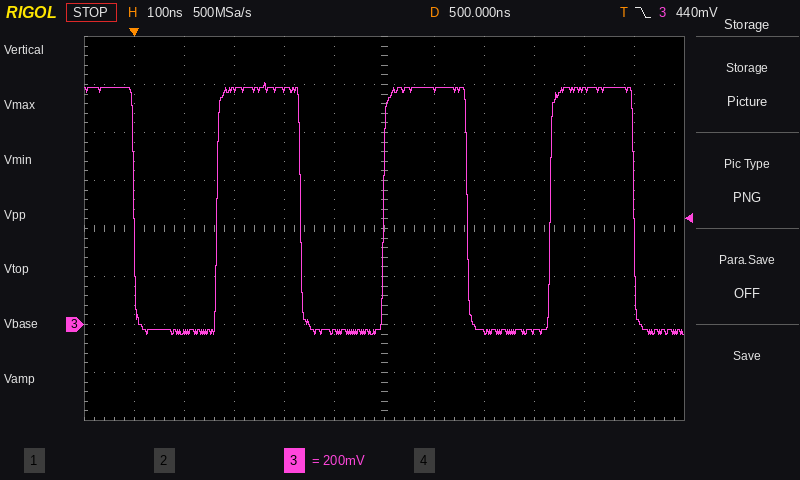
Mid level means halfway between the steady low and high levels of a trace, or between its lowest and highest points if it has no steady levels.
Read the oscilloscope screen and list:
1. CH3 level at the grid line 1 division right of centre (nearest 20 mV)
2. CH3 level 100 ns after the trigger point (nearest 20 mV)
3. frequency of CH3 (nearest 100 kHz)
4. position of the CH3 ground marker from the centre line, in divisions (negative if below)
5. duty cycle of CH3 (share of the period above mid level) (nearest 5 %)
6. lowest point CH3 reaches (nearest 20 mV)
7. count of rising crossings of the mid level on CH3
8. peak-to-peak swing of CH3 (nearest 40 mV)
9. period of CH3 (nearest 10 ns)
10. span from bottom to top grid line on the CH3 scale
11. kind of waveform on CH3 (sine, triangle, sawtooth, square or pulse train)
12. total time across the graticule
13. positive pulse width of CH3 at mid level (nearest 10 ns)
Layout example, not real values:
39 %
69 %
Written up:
980 mV
-40 mV
3.0 MHz
-2.0 div
50 %
-40 mV
3
1.04 V
330 ns
1.6 V
square
1.2 µs
170 ns
